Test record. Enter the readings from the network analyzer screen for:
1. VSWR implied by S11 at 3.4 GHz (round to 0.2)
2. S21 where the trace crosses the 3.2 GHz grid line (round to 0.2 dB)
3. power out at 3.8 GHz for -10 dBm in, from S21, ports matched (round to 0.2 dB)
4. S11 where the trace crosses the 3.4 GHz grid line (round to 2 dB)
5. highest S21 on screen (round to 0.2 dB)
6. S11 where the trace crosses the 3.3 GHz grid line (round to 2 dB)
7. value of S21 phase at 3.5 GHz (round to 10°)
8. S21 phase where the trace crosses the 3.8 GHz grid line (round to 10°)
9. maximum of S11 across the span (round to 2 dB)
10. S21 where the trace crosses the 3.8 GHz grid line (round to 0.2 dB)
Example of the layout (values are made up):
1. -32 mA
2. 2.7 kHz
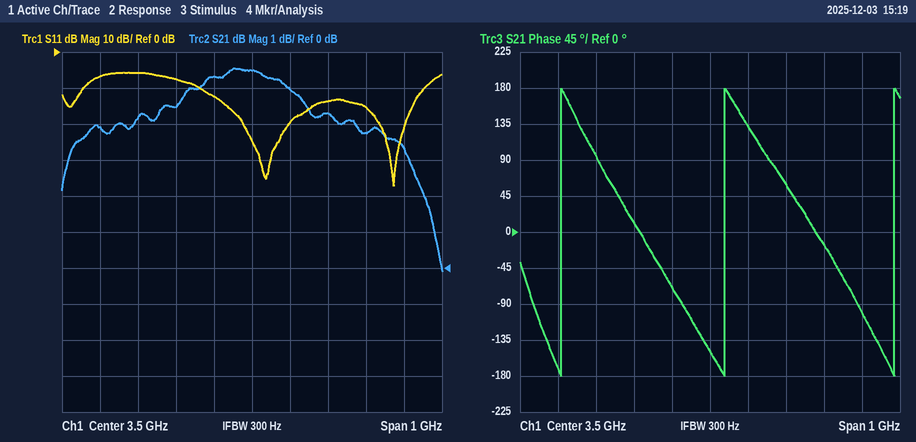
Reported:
1. 1.6
2. 4.2 dB
3. -6.2 dBm
4. -12 dB
5. 5.6 dB
6. -8 dB
7. -150°
8. -20°
9. -6 dB
10. 3.8 dB
